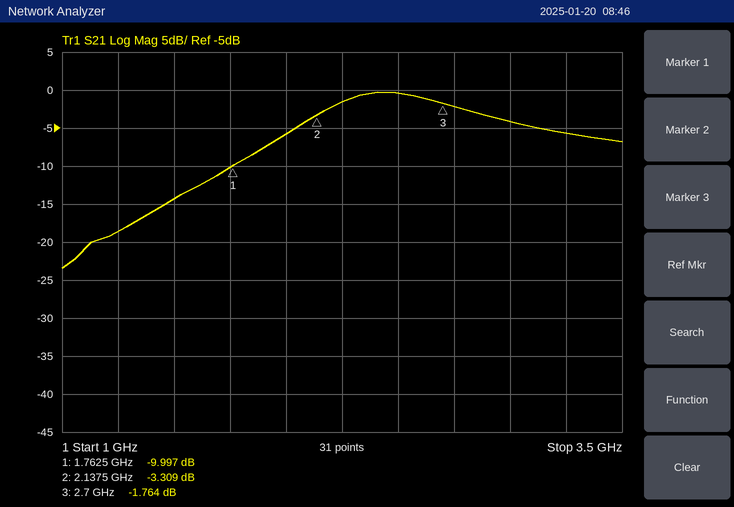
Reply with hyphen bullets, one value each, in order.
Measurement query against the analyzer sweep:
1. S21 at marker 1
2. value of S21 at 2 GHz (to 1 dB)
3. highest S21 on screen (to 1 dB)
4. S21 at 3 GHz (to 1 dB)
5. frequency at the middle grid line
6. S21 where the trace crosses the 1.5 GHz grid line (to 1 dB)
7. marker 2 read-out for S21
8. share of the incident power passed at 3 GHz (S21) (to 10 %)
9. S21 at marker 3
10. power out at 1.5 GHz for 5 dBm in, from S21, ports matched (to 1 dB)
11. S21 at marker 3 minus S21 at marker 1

- -9.997 dB
- -6 dB
- 0 dB
- -4 dB
- 2.25 GHz
- -14 dB
- -3.309 dB
- 40 %
- -1.764 dB
- -9 dBm
- 8.233 dB
